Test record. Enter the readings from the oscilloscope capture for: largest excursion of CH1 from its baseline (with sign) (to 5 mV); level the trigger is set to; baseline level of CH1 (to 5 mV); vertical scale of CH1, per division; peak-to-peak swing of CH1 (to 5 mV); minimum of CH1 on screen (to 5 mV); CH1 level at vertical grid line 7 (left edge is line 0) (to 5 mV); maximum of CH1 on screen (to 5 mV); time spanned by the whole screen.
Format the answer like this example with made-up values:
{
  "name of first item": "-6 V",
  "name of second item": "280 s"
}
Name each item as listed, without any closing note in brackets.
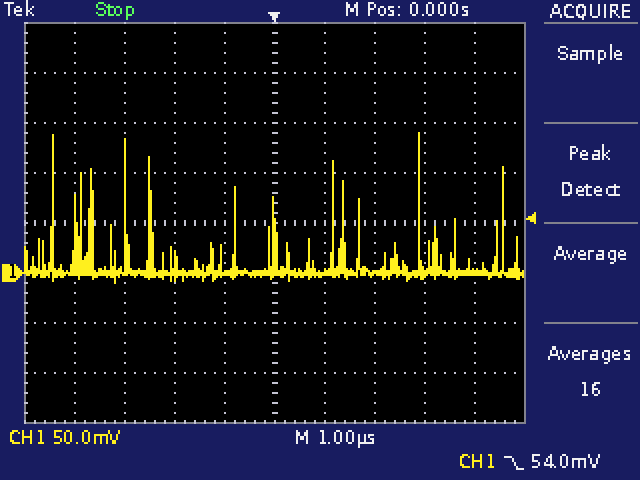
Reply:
{
  "largest excursion of CH1 from its baseline (with sign)": "+140 mV",
  "level the trigger is set to": "54.0 mV",
  "baseline level of CH1": "0 mV",
  "vertical scale of CH1, per division": "50 mV",
  "peak-to-peak swing of CH1": "150 mV",
  "minimum of CH1 on screen": "-10 mV",
  "CH1 level at vertical grid line 7 (left edge is line 0)": "0 mV",
  "maximum of CH1 on screen": "140 mV",
  "time spanned by the whole screen": "10 µs"
}
